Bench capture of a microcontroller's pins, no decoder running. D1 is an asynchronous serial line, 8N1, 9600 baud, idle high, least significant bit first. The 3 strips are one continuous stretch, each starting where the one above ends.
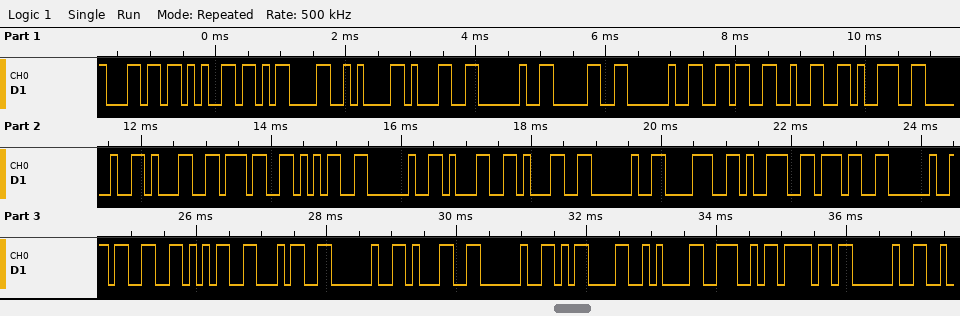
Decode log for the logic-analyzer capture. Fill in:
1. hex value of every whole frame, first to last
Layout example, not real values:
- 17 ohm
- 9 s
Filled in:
- 6C 65 0D 0A 31 20 30 20 36 32 39 20 31 37 35 20 31 31 20 38 39 37 20 33 35 34 20 31 20 0D 0A 4E 6F 20
